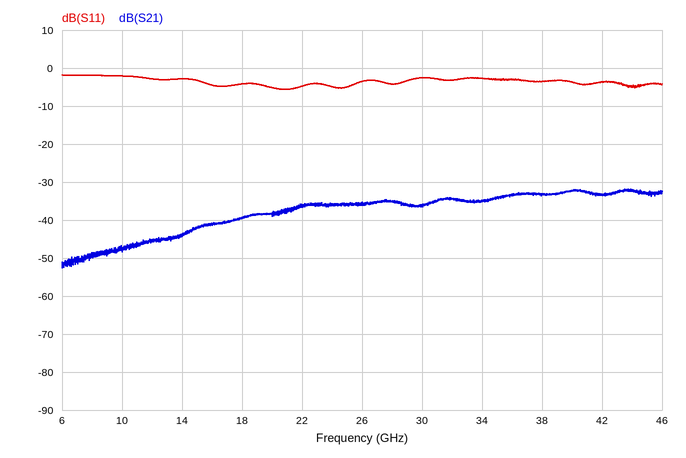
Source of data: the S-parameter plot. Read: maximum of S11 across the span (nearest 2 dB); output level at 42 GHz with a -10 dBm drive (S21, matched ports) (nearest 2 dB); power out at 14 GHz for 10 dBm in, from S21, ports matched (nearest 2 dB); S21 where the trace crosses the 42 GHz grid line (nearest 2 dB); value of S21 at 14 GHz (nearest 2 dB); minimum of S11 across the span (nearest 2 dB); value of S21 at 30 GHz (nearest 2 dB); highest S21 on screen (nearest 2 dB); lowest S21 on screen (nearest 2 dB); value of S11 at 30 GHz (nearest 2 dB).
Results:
-2 dB
-44 dBm
-34 dBm
-34 dB
-44 dB
-6 dB
-36 dB
-32 dB
-52 dB
-2 dB
